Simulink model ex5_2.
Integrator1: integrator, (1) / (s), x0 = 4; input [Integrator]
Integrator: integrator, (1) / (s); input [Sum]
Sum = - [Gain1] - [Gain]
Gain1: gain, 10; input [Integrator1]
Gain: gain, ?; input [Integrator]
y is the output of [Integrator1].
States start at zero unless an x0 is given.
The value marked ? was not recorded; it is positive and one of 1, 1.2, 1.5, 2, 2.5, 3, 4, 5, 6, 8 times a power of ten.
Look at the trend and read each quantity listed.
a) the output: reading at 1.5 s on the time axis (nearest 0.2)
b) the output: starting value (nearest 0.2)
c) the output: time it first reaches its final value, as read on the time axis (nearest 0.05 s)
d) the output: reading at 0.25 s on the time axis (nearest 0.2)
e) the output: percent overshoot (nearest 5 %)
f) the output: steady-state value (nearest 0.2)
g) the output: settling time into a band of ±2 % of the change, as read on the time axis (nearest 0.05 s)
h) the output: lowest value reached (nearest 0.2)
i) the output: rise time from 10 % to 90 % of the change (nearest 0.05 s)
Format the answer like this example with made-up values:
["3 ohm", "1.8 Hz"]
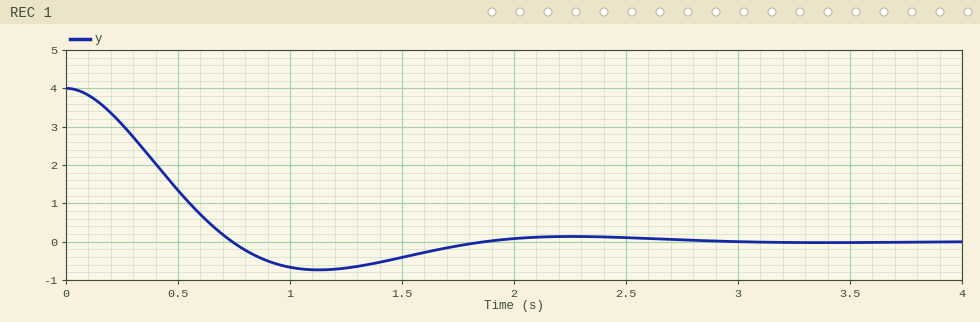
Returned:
["-0.4", "4.0", "0.75 s", "3.0", "20 %", "0.0", "2.60 s", "-0.8", "0.50 s"]
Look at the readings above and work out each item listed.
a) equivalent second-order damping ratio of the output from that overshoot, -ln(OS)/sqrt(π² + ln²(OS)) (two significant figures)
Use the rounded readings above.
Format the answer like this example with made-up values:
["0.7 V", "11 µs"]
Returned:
["0.46"]
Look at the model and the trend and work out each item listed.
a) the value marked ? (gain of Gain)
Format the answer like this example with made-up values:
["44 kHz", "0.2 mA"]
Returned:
["3"]
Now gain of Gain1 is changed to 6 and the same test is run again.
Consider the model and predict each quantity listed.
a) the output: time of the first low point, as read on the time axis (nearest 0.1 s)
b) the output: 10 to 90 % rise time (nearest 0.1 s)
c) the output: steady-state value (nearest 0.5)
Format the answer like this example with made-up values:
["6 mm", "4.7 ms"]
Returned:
["1.6 s", "0.8 s", "0.0"]
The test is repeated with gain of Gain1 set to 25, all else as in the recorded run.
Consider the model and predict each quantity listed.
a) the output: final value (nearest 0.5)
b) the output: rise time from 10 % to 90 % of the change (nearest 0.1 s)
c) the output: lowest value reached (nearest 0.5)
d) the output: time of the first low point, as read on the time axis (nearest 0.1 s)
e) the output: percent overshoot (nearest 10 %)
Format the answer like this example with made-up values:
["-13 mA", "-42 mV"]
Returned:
["0.0", "0.3 s", "-1.5", "0.7 s", "40 %"]
